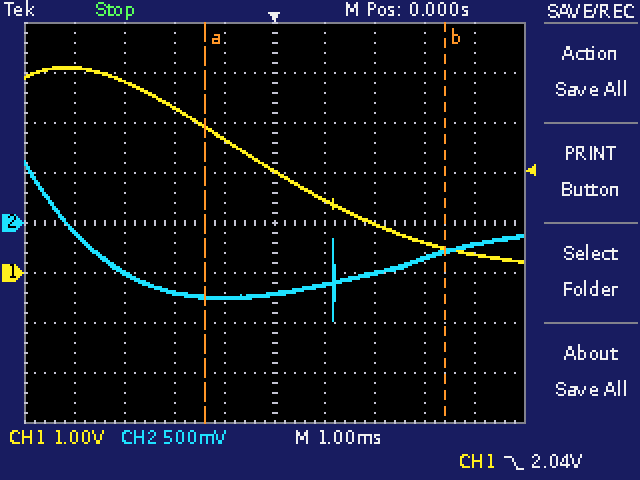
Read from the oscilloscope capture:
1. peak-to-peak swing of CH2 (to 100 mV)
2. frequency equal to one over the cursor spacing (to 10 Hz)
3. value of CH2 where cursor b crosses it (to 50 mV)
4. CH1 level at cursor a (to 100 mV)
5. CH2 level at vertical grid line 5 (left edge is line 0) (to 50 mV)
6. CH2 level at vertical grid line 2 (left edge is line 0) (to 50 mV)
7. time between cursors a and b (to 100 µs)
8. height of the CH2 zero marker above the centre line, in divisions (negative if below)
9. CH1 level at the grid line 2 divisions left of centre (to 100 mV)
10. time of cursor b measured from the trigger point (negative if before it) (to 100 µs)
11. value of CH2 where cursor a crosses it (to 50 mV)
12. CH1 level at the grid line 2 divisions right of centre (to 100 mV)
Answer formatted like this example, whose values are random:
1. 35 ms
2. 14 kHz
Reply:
1. 1.60 V
2. 210 Hz
3. -300 mV
4. 2.9 V
5. -700 mV
6. -500 mV
7. 4.8 ms
8. 0.0 div
9. 3.3 V
10. +3.4 ms
11. -750 mV
12. 1.0 V
